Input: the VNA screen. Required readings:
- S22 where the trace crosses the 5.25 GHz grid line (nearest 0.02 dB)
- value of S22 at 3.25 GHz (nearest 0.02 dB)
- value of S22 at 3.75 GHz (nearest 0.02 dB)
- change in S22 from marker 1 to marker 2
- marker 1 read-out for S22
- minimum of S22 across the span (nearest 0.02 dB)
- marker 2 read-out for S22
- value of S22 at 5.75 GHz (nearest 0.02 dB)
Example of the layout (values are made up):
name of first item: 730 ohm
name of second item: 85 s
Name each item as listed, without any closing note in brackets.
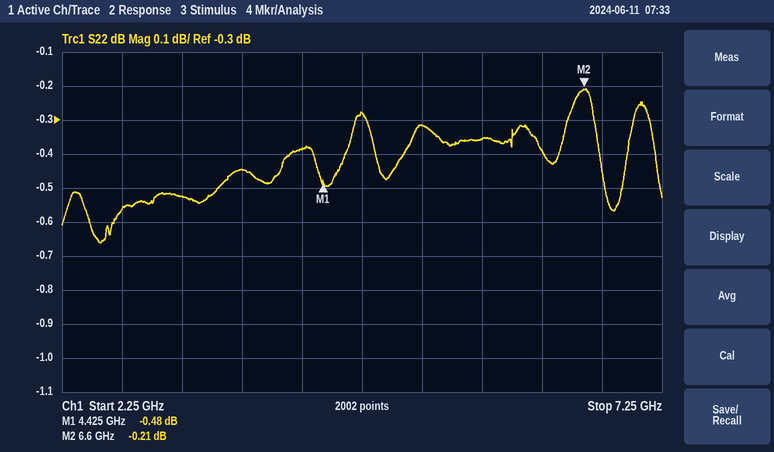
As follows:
S22 where the trace crosses the 5.25 GHz grid line: -0.32 dB
value of S22 at 3.25 GHz: -0.52 dB
value of S22 at 3.75 GHz: -0.44 dB
change in S22 from marker 1 to marker 2: 0.27 dB
marker 1 read-out for S22: -0.48 dB
minimum of S22 across the span: -0.66 dB
marker 2 read-out for S22: -0.21 dB
value of S22 at 5.75 GHz: -0.36 dB
